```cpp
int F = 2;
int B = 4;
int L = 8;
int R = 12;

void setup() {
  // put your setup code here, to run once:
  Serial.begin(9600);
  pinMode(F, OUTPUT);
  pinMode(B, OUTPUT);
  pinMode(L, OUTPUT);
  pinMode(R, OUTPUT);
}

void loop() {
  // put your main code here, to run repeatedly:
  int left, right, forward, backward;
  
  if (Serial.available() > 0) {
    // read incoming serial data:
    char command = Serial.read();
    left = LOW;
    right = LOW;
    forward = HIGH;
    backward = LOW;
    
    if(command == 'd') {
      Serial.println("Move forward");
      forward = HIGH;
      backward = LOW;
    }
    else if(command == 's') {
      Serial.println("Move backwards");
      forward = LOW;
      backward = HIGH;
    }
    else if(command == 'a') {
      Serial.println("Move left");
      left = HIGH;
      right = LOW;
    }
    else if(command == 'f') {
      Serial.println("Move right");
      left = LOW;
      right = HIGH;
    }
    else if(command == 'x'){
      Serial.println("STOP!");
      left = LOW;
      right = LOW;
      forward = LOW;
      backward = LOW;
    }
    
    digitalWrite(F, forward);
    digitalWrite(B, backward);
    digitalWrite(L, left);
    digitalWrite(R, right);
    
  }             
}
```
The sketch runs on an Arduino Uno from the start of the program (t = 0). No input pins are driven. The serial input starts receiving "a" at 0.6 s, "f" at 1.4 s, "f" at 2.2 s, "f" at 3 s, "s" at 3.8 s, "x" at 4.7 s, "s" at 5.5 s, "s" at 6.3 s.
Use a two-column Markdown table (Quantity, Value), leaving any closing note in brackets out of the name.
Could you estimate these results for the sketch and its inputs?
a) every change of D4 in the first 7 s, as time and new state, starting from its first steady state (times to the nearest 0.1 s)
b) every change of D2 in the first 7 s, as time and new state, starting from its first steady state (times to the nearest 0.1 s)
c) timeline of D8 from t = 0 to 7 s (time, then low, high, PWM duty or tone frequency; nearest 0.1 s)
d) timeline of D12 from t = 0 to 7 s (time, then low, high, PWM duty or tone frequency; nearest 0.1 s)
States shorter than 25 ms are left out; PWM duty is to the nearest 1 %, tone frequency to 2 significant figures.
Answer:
| Quantity | Value |
|---|---|
| every change of D4 in the first 7 s, as time and new state, starting from its first steady state | 0 s low; 3.8 s high; 4.7 s low; 5.5 s high |
| every change of D2 in the first 7 s, as time and new state, starting from its first steady state | 0 s low; 0.6 s high; 3.8 s low |
| timeline of D8 from t = 0 to 7 s | 0 s low; 0.6 s high; 1.4 s low |
| timeline of D12 from t = 0 to 7 s | 0 s low; 1.4 s high; 3.8 s low |
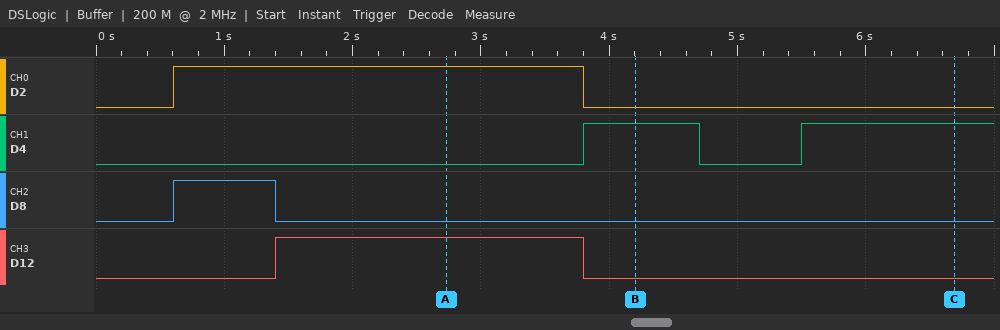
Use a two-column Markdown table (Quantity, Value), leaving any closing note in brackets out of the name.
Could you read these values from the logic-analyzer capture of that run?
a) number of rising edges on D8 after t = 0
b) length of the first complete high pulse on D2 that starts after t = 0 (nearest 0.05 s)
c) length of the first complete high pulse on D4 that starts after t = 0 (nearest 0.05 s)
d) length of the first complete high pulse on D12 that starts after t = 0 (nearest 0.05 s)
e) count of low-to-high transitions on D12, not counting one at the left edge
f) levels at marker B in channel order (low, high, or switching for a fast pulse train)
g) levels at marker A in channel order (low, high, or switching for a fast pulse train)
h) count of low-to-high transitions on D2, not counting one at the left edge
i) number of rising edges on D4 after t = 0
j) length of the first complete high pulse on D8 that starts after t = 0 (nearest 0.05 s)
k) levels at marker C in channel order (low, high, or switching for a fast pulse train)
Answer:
| Quantity | Value |
|---|---|
| number of rising edges on D8 after t = 0 | 1 |
| length of the first complete high pulse on D2 that starts after t = 0 | 3.20 s |
| length of the first complete high pulse on D4 that starts after t = 0 | 0.90 s |
| length of the first complete high pulse on D12 that starts after t = 0 | 2.40 s |
| count of low-to-high transitions on D12, not counting one at the left edge | 1 |
| levels at marker B in channel order | D2 low, D4 high, D8 low, D12 low |
| levels at marker A in channel order | D2 high, D4 low, D8 low, D12 high |
| count of low-to-high transitions on D2, not counting one at the left edge | 1 |
| number of rising edges on D4 after t = 0 | 2 |
| length of the first complete high pulse on D8 that starts after t = 0 | 0.80 s |
| levels at marker C in channel order | D2 low, D4 high, D8 low, D12 low |
